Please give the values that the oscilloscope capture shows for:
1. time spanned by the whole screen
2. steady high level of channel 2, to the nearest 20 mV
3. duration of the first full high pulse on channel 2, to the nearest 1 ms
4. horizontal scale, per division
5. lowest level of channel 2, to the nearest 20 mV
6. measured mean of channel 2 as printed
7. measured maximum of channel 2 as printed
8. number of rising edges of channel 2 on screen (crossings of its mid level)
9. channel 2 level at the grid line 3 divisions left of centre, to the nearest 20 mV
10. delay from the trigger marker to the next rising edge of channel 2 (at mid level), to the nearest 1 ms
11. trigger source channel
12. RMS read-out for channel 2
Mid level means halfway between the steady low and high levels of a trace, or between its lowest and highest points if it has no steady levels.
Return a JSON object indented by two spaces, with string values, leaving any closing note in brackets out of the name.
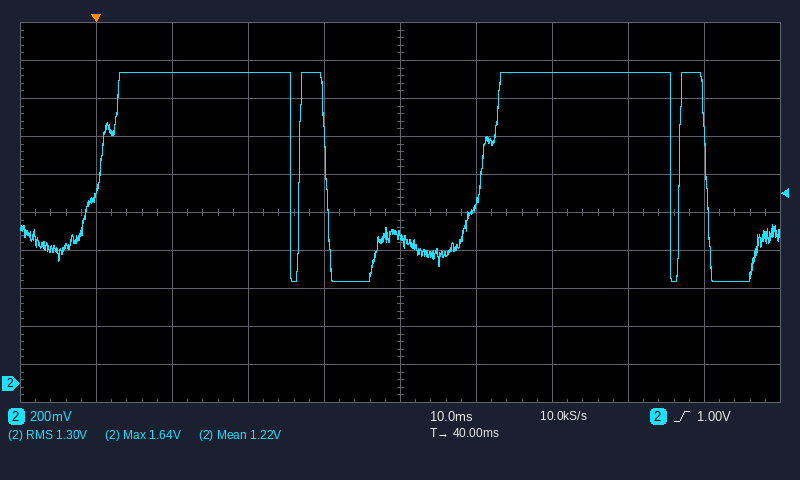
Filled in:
{
  "time spanned by the whole screen": "100 ms",
  "steady high level of channel 2, to the nearest 20 mV": "1.64 V",
  "duration of the first full high pulse on channel 2, to the nearest 1 ms": "25 ms",
  "horizontal scale, per division": "10 ms",
  "lowest level of channel 2, to the nearest 20 mV": "540 mV",
  "measured mean of channel 2 as printed": "1.22 V",
  "measured maximum of channel 2 as printed": "1.64 V",
  "number of rising edges of channel 2 on screen": "4",
  "channel 2 level at the grid line 3 divisions left of centre, to the nearest 20 mV": "1.64 V",
  "delay from the trigger marker to the next rising edge of channel 2 (at mid level), to the nearest 1 ms": "27 ms",
  "trigger source channel": "channel 2",
  "RMS read-out for channel 2": "1.30 V"
}
